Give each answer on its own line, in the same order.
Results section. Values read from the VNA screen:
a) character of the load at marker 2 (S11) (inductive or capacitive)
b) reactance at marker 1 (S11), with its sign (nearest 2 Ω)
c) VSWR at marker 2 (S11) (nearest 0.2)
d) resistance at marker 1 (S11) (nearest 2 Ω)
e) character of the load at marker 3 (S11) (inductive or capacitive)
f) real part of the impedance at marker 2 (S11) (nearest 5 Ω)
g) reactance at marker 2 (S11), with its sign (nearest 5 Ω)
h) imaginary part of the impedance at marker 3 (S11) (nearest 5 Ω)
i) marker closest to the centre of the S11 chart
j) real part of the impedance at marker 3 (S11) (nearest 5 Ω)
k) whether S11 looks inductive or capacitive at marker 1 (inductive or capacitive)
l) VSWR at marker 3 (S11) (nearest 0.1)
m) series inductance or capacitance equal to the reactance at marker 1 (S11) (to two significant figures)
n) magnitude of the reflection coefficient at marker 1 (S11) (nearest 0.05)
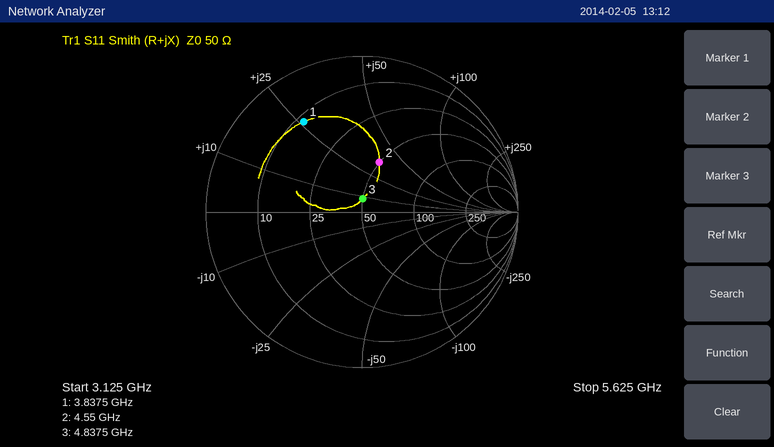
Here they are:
inductive
+26 Ω
2.0
12 Ω
inductive
50 Ω
+35 Ω
+10 Ω
marker 3
50 Ω
inductive
1.2
1.1 nH
0.70
